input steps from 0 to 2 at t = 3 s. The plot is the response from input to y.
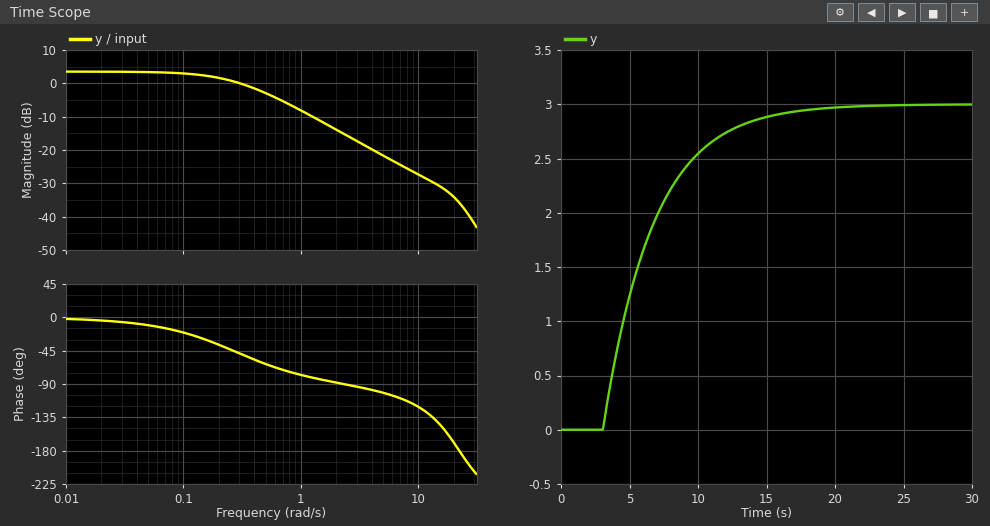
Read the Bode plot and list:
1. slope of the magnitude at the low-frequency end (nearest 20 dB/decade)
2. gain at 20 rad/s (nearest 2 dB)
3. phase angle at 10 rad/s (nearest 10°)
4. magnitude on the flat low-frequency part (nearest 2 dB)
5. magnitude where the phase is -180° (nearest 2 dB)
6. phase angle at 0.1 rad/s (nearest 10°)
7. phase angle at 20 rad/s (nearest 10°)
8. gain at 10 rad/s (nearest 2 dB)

0 dB/decade
-34 dB
-120°
4 dB
-36 dB
-20°
-170°
-28 dB
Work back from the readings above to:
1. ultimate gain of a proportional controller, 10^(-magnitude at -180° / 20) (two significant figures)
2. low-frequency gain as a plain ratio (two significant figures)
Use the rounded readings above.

63
1.6
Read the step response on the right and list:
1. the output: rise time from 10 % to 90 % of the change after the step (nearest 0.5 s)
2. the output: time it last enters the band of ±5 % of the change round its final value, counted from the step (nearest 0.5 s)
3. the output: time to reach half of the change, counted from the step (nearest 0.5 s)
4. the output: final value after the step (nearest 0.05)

8.0 s
11.0 s
2.5 s
3.00
